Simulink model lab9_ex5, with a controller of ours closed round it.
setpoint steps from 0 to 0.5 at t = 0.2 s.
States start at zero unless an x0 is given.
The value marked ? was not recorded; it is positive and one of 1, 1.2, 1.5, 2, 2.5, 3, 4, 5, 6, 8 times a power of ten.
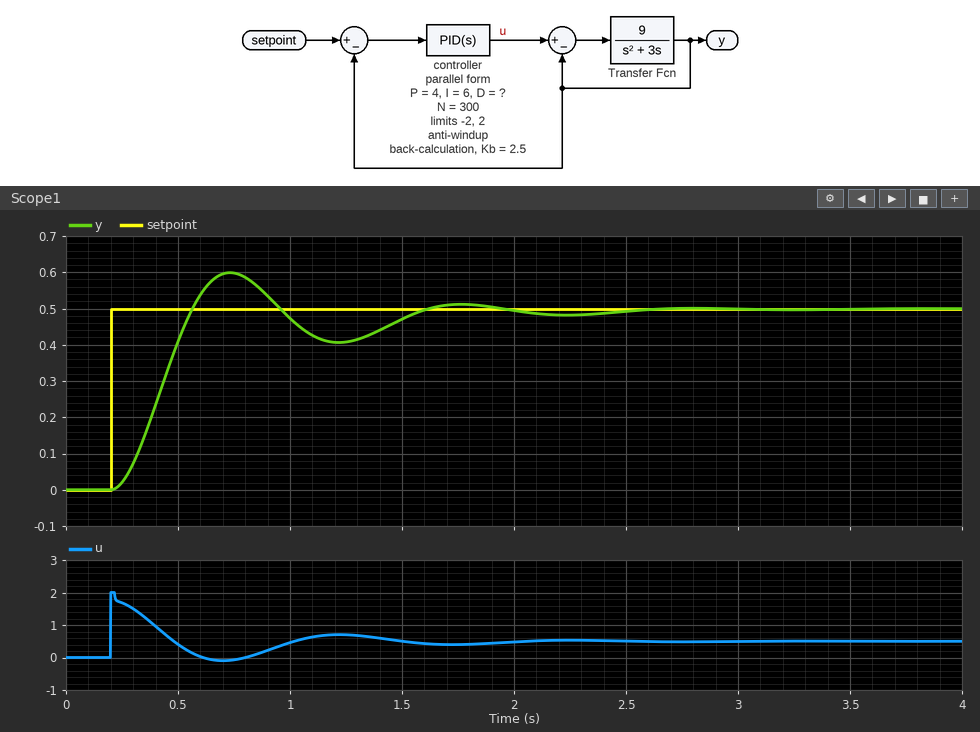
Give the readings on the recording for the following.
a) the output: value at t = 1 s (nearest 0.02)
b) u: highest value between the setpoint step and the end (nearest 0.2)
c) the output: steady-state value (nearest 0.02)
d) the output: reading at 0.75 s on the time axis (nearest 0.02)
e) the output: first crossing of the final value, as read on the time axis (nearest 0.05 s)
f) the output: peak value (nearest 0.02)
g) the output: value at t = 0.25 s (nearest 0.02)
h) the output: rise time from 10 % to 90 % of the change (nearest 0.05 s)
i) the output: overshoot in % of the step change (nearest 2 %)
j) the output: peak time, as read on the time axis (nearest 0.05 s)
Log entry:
0.48
2.0
0.50
0.60
0.55 s
0.60
0.02
0.25 s
20 %
0.75 s
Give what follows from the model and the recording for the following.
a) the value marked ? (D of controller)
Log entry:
0.2
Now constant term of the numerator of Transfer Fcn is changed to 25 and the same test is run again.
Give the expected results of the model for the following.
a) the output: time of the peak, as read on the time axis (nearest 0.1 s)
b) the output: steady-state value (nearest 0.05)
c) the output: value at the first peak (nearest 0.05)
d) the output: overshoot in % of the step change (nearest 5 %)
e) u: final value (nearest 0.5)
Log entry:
0.5 s
0.50
0.55
10 %
0.5
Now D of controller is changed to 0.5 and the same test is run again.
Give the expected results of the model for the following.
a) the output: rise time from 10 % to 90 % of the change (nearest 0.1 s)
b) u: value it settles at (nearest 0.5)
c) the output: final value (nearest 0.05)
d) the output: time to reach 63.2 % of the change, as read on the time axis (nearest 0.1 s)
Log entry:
0.4 s
0.5
0.50
0.5 s
